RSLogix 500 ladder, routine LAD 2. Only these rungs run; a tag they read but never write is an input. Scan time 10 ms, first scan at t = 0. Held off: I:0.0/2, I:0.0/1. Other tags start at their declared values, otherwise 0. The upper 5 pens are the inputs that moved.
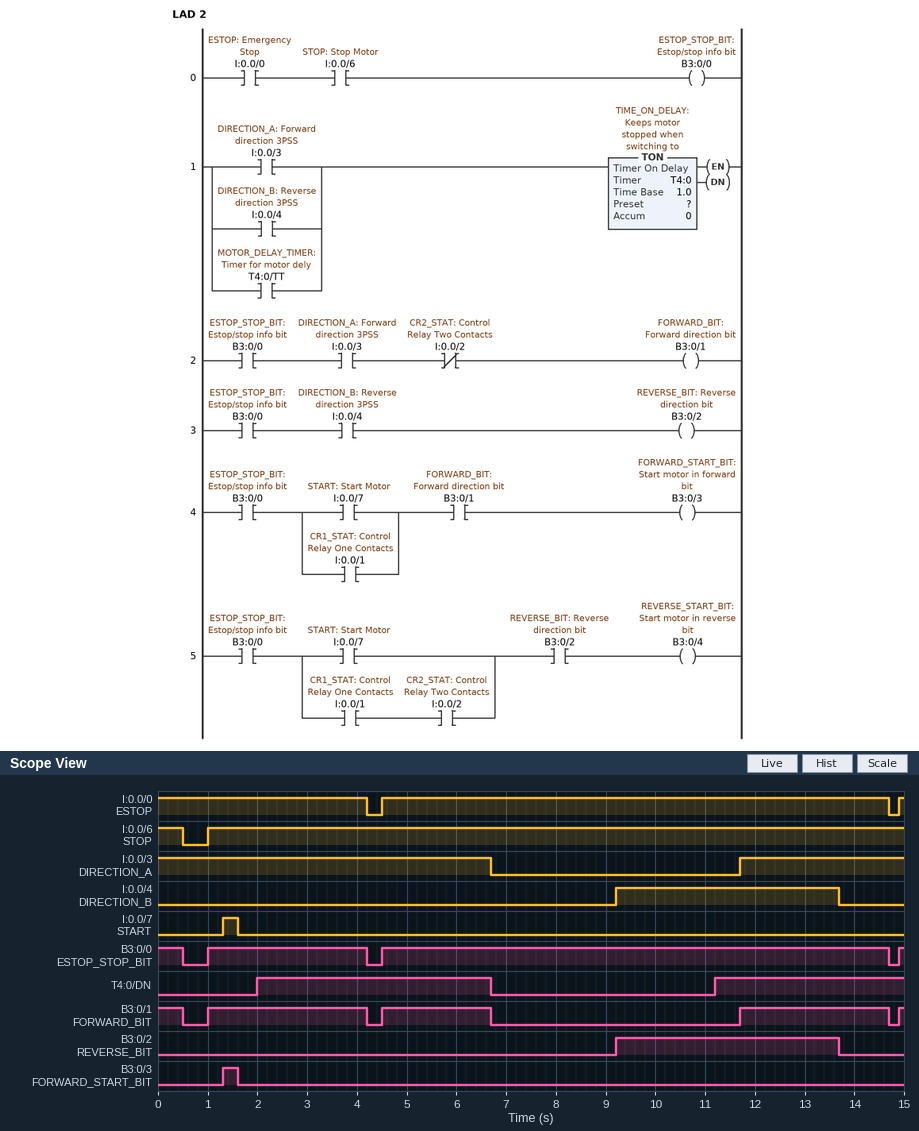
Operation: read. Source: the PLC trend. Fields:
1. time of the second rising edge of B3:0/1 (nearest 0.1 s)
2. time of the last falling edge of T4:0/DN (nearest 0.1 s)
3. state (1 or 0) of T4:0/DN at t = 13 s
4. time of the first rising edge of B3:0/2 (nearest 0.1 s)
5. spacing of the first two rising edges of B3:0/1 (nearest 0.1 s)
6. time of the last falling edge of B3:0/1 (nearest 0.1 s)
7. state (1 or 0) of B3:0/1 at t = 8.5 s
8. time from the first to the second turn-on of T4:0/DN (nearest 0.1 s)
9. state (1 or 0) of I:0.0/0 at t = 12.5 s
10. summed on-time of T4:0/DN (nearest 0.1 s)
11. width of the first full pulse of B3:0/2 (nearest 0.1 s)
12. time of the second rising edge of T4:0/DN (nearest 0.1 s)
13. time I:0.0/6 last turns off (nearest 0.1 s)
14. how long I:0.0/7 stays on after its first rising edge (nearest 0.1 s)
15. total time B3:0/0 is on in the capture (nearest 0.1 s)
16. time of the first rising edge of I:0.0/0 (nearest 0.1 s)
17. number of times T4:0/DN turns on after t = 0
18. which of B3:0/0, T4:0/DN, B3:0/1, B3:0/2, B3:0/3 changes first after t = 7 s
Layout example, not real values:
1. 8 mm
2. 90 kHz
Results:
1. 4.5 s
2. 6.7 s
3. 1
4. 9.2 s
5. 3.5 s
6. 14.7 s
7. 0
8. 9.2 s
9. 1
10. 8.5 s
11. 4.5 s
12. 11.2 s
13. 0.5 s
14. 0.3 s
15. 14.0 s
16. 4.5 s
17. 2
18. B3:0/2
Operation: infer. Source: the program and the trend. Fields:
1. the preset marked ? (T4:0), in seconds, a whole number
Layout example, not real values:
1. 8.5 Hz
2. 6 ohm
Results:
1. 2 s
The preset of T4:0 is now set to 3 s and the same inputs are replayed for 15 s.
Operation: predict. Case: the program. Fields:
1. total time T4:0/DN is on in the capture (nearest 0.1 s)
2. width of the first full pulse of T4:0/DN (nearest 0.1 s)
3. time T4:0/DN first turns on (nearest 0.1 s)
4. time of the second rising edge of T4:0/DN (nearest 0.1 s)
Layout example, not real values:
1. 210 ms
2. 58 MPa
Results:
1. 6.5 s
2. 3.7 s
3. 3.0 s
4. 12.2 s
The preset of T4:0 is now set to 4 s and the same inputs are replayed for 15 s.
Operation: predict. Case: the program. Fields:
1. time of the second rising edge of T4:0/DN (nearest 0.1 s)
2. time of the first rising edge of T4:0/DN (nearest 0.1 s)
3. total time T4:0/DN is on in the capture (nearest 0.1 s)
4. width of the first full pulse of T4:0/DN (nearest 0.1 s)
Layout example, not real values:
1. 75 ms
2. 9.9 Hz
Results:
1. 13.2 s
2. 4.0 s
3. 4.5 s
4. 2.7 s
